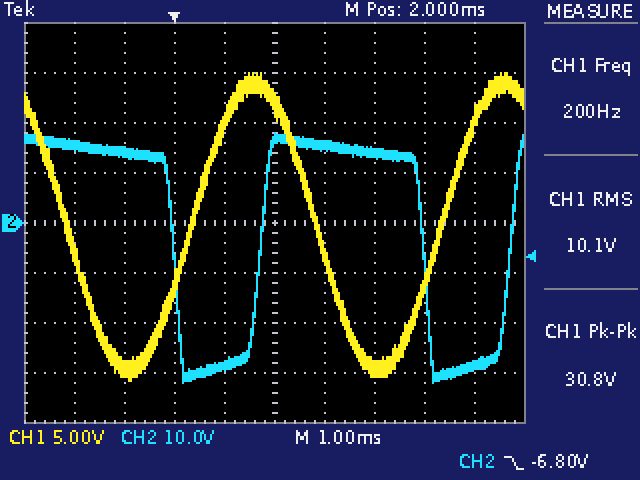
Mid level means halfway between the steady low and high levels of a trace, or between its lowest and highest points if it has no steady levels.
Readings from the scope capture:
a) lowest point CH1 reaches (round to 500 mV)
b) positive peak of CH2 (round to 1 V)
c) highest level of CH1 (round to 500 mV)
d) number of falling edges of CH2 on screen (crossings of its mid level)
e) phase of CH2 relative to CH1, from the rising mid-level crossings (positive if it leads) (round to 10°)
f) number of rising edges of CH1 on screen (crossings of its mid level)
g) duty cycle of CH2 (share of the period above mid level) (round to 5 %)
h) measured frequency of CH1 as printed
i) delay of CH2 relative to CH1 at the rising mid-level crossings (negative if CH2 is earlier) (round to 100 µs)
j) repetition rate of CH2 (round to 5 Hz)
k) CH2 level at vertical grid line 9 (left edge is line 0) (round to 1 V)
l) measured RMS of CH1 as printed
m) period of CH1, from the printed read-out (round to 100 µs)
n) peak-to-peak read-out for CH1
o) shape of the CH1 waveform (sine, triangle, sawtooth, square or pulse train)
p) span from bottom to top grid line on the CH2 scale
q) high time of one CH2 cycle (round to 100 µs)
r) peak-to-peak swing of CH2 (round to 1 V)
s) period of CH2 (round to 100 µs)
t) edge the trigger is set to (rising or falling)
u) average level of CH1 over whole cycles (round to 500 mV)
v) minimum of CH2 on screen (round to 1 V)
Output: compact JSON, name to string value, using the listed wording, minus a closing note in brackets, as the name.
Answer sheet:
{"lowest point CH1 reaches": "-16.0 V", "positive peak of CH2": "18 V", "highest level of CH1": "15.0 V", "number of falling edges of CH2 on screen": "2", "phase of CH2 relative to CH1, from the rising mid-level crossings (positive if it leads)": "-100°", "number of rising edges of CH1 on screen": "2", "duty cycle of CH2 (share of the period above mid level)": "65 %", "measured frequency of CH1 as printed": "200 Hz", "delay of CH2 relative to CH1 at the rising mid-level crossings (negative if CH2 is earlier)": "+1.4 ms", "repetition rate of CH2": "200 Hz", "CH2 level at vertical grid line 9 (left edge is line 0)": "-29 V", "measured RMS of CH1 as printed": "10.1 V", "period of CH1, from the printed read-out": "5.0 ms", "peak-to-peak read-out for CH1": "30.8 V", "shape of the CH1 waveform": "sine", "span from bottom to top grid line on the CH2 scale": "80 V", "high time of one CH2 cycle": "3.3 ms", "peak-to-peak swing of CH2": "50 V", "period of CH2": "5.0 ms", "edge the trigger is set to": "falling", "average level of CH1 over whole cycles": "-500 mV", "minimum of CH2 on screen": "-32 V"}
